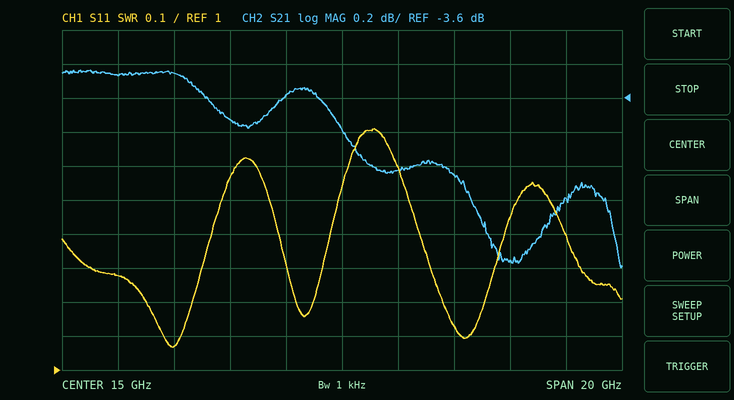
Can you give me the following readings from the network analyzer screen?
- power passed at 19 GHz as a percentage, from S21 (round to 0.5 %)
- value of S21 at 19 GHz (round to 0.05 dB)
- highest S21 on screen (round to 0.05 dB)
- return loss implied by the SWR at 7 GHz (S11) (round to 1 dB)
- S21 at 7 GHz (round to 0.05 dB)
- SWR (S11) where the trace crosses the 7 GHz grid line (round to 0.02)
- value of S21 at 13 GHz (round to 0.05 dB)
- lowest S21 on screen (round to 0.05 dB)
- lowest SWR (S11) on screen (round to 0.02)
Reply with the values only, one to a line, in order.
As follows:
39.5 %
-4.05 dB
-3.45 dB
18 dB
-3.45 dB
1.28
-3.60 dB
-4.60 dB
1.06
